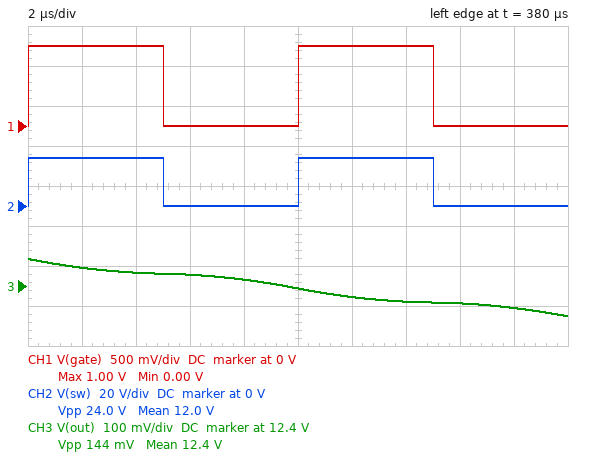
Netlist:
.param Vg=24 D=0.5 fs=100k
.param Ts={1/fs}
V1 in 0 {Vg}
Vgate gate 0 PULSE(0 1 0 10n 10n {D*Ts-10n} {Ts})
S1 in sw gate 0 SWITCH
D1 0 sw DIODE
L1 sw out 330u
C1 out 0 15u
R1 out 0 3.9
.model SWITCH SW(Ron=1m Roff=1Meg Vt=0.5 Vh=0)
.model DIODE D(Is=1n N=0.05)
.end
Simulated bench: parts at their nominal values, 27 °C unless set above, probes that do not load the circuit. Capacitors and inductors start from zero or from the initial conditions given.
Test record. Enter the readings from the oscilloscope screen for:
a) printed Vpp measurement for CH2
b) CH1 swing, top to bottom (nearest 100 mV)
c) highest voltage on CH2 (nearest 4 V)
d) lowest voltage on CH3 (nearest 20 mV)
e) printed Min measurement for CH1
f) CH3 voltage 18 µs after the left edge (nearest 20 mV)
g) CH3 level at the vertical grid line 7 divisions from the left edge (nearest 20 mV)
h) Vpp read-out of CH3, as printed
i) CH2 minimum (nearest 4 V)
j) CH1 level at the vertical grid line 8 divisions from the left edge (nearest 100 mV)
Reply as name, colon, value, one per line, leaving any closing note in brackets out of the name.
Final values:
printed Vpp measurement for CH2: 24.0 V
CH1 swing, top to bottom: 1.0 V
highest voltage on CH2: 24 V
lowest voltage on CH3: 12.32 V
printed Min measurement for CH1: 0.00 V
CH3 voltage 18 µs after the left edge: 12.34 V
CH3 level at the vertical grid line 7 divisions from the left edge: 12.36 V
Vpp read-out of CH3, as printed: 144 mV
CH2 minimum: 0 V
CH1 level at the vertical grid line 8 divisions from the left edge: 0 V
